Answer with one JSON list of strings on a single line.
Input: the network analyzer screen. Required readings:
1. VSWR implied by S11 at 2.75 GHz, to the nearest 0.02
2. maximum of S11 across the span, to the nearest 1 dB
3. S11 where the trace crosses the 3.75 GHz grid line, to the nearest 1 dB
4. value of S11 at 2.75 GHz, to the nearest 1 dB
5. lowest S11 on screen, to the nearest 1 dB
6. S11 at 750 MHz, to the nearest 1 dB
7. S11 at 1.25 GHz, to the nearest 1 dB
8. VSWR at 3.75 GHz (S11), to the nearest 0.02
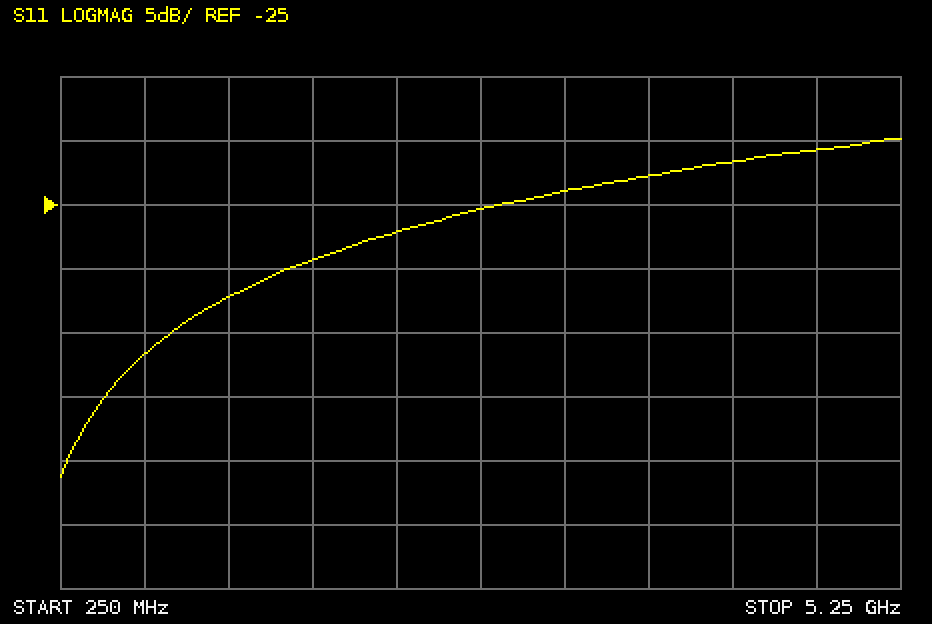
["1.12", "-20 dB", "-23 dB", "-25 dB", "-46 dB", "-37 dB", "-32 dB", "1.16"]
